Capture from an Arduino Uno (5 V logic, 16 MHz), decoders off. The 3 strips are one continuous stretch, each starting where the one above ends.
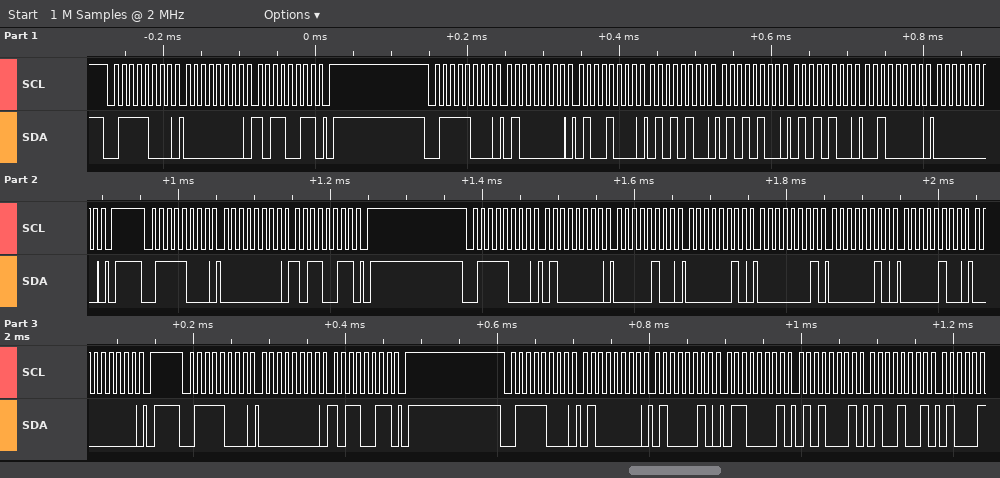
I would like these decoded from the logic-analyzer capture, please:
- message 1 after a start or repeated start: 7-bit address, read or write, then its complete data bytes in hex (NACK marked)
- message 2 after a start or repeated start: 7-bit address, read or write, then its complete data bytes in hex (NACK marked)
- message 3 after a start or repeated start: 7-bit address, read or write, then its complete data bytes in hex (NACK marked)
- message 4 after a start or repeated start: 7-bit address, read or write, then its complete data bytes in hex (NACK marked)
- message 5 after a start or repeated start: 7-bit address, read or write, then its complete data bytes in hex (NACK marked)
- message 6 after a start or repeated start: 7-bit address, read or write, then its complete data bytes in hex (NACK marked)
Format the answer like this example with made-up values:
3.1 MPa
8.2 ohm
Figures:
0x3C write: 00 B3
0x3C write: 40 48 54 54 54 20 00
0x3C write: 00 B3
0x3C write: 40 04 02 01 02 04 00
0x3C write: 00 B3
0x3C write: 40 42 61 51 49
